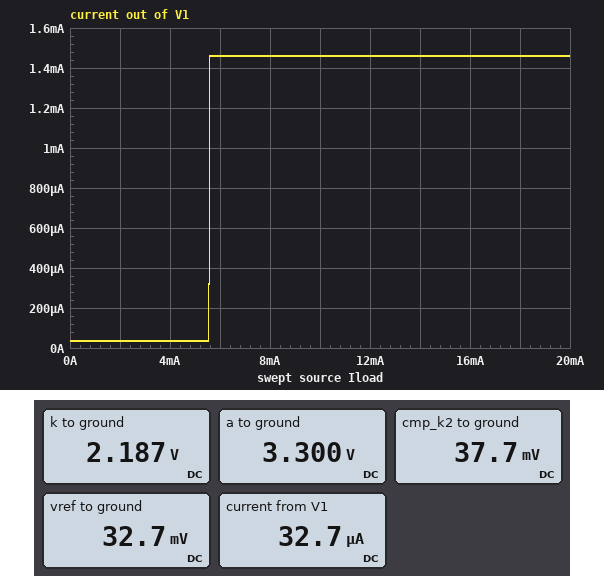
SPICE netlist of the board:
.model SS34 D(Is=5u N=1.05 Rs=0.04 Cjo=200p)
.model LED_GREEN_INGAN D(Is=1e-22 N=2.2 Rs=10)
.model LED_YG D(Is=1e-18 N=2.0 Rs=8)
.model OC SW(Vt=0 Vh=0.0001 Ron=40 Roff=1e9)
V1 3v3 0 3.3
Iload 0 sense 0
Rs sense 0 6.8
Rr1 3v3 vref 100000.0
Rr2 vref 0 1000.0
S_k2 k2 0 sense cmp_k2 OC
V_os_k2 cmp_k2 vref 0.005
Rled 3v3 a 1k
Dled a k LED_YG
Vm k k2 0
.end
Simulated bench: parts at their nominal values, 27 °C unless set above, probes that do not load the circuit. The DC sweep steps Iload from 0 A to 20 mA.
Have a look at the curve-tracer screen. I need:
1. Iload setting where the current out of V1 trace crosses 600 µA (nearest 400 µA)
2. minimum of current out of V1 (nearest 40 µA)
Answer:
5.6 mA
40 µA
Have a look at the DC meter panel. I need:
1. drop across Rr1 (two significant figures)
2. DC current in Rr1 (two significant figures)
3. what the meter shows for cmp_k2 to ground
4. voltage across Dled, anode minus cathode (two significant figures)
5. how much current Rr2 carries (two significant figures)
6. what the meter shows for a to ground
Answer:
3.3 V
33 µA
37.7 mV
1.1 V
33 µA
3.300 V
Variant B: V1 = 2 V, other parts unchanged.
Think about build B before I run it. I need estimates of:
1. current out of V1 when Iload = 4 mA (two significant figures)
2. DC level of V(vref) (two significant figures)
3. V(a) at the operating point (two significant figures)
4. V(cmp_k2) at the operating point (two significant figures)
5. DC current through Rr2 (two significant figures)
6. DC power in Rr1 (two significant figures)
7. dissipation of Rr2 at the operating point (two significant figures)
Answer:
290 µA
20 mV
2.0 V
25 mV
20 µA
39 µW
390 nW
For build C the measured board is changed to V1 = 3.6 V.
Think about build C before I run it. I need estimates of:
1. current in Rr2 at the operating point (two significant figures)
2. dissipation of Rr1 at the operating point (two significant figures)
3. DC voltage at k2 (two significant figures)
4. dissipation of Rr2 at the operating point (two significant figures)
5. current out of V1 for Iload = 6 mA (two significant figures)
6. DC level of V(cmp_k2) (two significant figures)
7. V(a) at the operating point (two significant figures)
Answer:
36 µA
130 µW
2.5 V
1.3 µW
1.7 mA
41 mV
3.6 V
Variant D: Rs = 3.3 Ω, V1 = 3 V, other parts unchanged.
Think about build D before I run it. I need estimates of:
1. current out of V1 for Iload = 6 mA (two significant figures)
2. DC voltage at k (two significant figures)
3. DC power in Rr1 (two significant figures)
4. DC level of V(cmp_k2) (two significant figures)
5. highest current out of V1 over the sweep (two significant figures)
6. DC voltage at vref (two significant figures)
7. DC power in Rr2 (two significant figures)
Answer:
30 µA
1.9 V
88 µW
35 mV
1.2 mA
30 mV
880 nW
